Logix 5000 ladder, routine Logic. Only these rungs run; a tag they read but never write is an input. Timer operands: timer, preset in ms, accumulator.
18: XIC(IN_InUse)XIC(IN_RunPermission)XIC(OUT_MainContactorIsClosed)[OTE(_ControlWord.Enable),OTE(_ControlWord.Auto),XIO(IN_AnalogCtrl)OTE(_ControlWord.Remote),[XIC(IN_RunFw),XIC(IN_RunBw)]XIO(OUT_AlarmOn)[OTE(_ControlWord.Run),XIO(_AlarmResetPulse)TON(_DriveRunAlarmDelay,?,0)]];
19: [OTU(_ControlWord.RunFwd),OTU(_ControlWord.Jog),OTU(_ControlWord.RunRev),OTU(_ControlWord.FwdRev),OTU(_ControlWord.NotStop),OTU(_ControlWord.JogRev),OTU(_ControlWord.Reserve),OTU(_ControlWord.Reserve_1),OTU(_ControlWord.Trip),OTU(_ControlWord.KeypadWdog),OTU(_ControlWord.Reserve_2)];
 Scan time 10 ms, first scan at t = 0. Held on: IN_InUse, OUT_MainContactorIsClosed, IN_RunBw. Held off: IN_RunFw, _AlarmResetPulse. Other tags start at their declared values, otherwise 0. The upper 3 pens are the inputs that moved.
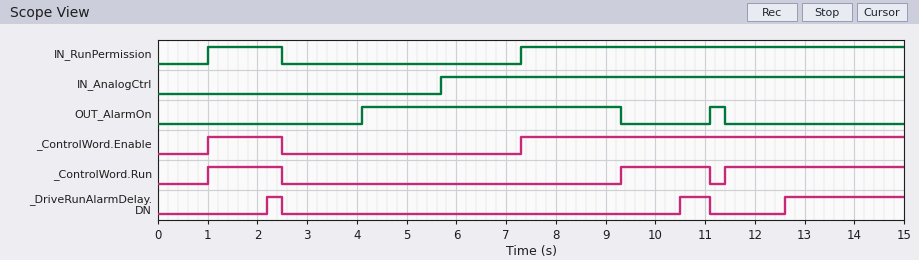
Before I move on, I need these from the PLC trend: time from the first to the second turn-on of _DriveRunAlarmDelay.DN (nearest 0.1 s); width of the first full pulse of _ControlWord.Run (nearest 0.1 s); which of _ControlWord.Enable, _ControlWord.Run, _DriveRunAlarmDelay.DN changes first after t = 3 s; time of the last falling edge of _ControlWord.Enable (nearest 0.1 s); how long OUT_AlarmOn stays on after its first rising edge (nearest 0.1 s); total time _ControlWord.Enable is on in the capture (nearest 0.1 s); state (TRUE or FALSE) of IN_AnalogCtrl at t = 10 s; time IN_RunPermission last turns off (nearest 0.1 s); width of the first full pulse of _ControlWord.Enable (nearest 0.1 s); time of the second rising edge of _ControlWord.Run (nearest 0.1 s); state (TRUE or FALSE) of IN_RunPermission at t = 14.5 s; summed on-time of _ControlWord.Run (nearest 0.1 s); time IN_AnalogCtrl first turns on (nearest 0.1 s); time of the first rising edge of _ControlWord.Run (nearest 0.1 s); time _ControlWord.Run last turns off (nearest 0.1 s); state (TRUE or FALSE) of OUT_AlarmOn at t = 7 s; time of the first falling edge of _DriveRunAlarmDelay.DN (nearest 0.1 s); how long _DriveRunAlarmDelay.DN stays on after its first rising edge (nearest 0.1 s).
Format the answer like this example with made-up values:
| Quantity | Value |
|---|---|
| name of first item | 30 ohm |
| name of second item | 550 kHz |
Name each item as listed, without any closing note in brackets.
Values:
| Quantity | Value |
|---|---|
| time from the first to the second turn-on of _DriveRunAlarmDelay.DN | 8.3 s |
| width of the first full pulse of _ControlWord.Run | 1.5 s |
| which of _ControlWord.Enable, _ControlWord.Run, _DriveRunAlarmDelay.DN changes first after t = 3 s | _ControlWord.Enable |
| time of the last falling edge of _ControlWord.Enable | 2.5 s |
| how long OUT_AlarmOn stays on after its first rising edge | 5.2 s |
| total time _ControlWord.Enable is on in the capture | 9.2 s |
| state (TRUE or FALSE) of IN_AnalogCtrl at t = 10 s | TRUE |
| time IN_RunPermission last turns off | 2.5 s |
| width of the first full pulse of _ControlWord.Enable | 1.5 s |
| time of the second rising edge of _ControlWord.Run | 9.3 s |
| state (TRUE or FALSE) of IN_RunPermission at t = 14.5 s | TRUE |
| summed on-time of _ControlWord.Run | 6.9 s |
| time IN_AnalogCtrl first turns on | 5.7 s |
| time of the first rising edge of _ControlWord.Run | 1.0 s |
| time _ControlWord.Run last turns off | 11.1 s |
| state (TRUE or FALSE) of OUT_AlarmOn at t = 7 s | TRUE |
| time of the first falling edge of _DriveRunAlarmDelay.DN | 2.5 s |
| how long _DriveRunAlarmDelay.DN stays on after its first rising edge | 0.3 s |
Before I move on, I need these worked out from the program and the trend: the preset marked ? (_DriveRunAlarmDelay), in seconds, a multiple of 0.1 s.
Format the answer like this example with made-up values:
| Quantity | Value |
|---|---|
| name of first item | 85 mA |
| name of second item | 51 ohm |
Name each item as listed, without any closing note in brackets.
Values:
| Quantity | Value |
|---|---|
| the preset marked ? (_DriveRunAlarmDelay), in seconds, a multiple of 0.1 s | 1.2 s |
